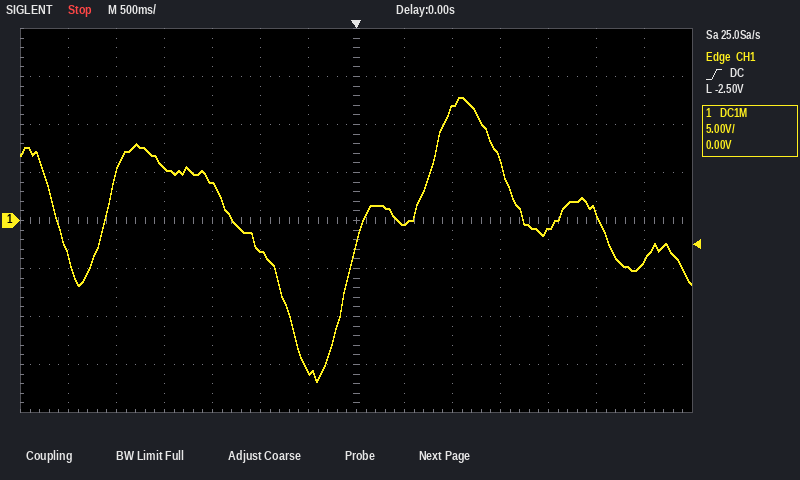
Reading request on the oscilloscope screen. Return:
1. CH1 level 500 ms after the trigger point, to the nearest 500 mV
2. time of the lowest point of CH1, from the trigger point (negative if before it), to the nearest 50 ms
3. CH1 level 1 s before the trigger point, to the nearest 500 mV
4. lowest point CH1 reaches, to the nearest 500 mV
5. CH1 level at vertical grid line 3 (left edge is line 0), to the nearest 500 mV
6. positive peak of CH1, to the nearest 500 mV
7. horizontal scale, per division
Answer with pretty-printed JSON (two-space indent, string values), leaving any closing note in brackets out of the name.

{
  "CH1 level 500 ms after the trigger point, to the nearest 500 mV": "-500 mV",
  "time of the lowest point of CH1, from the trigger point (negative if before it), to the nearest 50 ms": "-400 ms",
  "CH1 level 1 s before the trigger point, to the nearest 500 mV": "-3.0 V",
  "lowest point CH1 reaches, to the nearest 500 mV": "-17.0 V",
  "CH1 level at vertical grid line 3 (left edge is line 0), to the nearest 500 mV": "5.5 V",
  "positive peak of CH1, to the nearest 500 mV": "13.0 V",
  "horizontal scale, per division": "500 ms"
}
